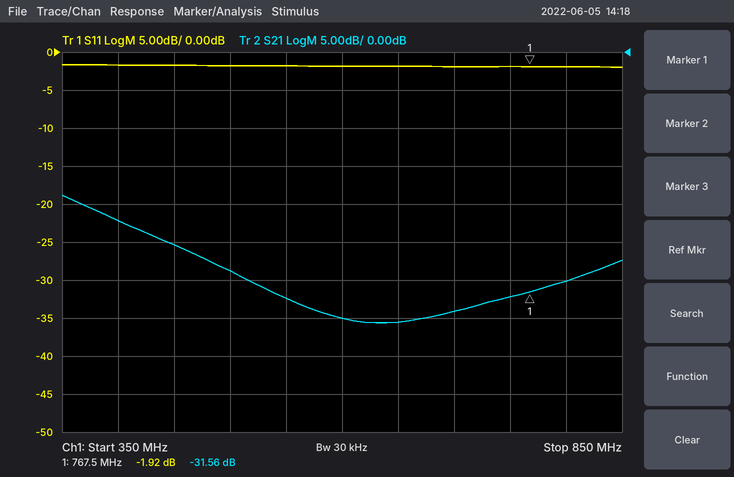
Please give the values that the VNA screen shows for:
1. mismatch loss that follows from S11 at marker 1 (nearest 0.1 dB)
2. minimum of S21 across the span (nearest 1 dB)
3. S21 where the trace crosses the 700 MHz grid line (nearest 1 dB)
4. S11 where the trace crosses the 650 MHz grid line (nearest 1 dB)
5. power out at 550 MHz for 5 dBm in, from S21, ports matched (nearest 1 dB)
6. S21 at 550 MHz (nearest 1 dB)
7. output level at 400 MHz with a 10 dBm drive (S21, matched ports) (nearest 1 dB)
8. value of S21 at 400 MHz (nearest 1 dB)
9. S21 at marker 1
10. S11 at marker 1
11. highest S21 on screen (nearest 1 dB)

4.5 dB
-36 dB
-34 dB
-2 dB
-27 dBm
-32 dB
-12 dBm
-22 dB
-31.56 dB
-1.92 dB
-19 dB
